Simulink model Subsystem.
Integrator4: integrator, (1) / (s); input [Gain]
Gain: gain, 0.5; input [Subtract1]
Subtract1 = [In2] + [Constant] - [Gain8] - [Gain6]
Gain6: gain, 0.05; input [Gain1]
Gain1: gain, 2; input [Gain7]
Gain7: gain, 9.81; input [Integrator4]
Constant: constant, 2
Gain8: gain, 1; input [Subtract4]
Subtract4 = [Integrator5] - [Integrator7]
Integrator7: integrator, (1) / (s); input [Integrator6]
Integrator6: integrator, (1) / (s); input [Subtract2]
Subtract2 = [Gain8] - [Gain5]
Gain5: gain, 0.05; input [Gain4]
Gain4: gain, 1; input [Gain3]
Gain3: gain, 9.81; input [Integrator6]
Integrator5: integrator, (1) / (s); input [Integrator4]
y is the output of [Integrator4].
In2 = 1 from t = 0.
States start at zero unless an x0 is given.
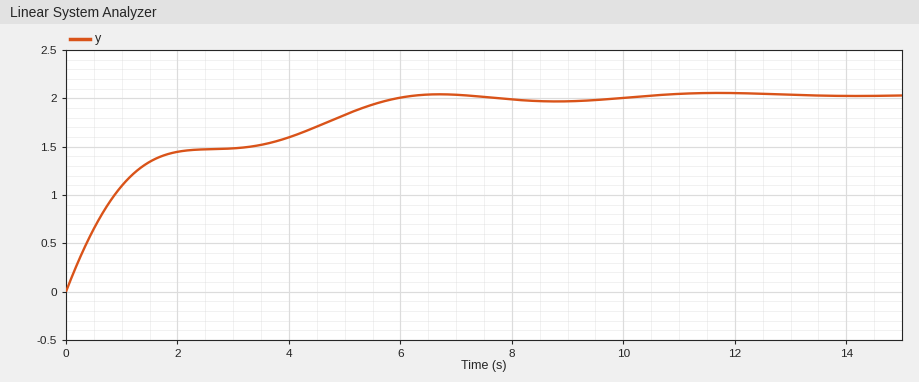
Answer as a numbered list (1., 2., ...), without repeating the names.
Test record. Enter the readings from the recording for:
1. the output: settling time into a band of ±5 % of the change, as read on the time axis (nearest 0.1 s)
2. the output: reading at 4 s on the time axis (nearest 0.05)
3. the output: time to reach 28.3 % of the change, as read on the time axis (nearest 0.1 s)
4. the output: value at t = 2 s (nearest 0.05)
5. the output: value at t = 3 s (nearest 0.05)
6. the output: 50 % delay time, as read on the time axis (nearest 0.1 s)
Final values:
1. 5.5 s
2. 1.60
3. 0.4 s
4. 1.45
5. 1.50
6. 0.9 s
